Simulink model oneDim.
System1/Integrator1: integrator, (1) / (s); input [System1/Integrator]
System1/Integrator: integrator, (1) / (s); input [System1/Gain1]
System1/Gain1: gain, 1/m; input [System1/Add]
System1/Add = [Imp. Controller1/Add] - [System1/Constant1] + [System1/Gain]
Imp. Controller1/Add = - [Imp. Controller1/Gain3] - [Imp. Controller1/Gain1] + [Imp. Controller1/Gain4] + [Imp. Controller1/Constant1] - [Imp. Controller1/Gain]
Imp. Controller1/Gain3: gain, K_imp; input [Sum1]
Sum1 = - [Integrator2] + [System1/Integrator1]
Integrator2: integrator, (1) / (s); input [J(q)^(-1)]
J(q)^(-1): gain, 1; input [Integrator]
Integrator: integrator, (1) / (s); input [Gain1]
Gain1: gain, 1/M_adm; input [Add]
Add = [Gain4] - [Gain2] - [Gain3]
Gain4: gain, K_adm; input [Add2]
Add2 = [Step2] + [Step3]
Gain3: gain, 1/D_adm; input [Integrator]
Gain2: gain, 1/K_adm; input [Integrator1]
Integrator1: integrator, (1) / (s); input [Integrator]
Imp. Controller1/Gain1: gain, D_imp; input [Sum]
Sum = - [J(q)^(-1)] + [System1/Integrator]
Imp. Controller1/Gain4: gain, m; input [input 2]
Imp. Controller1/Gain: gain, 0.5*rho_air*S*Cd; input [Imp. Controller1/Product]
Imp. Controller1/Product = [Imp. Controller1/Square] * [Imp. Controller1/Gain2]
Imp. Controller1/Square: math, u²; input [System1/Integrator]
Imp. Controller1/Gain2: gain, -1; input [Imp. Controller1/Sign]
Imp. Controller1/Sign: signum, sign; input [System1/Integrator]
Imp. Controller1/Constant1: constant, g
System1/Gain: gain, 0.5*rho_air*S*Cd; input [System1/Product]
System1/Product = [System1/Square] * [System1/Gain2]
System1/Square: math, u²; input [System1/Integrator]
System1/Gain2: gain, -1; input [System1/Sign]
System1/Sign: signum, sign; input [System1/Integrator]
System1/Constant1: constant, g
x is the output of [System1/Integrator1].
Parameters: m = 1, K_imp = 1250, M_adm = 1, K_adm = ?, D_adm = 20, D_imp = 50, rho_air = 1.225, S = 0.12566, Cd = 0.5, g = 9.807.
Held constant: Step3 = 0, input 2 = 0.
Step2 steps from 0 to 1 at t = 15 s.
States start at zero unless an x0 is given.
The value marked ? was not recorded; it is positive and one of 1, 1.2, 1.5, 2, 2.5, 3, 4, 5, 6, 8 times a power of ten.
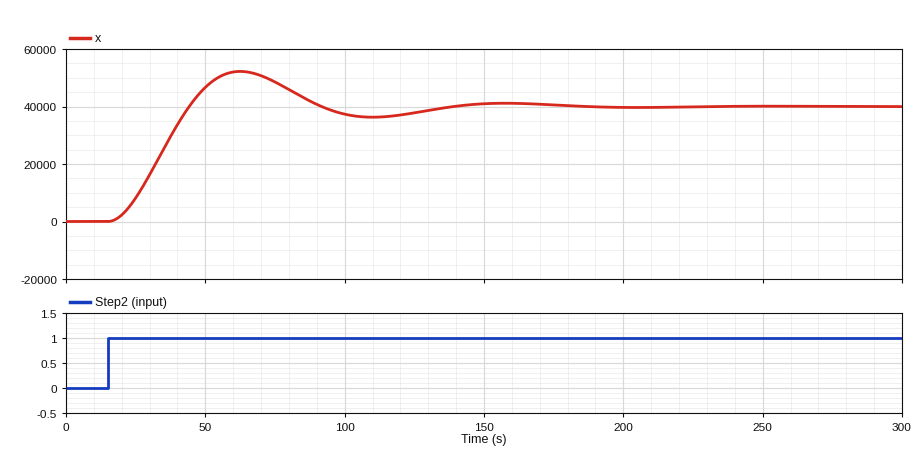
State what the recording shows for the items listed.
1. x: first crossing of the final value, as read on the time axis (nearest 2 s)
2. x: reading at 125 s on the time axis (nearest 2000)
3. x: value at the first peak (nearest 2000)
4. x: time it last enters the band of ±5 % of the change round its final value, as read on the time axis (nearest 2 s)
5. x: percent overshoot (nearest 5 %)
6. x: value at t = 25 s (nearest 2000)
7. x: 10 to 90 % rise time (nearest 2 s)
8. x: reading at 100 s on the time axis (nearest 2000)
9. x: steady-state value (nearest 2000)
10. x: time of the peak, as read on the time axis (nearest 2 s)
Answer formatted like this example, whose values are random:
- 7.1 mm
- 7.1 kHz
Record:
- 44 s
- 38000
- 52000
- 126 s
- 30 %
- 8000
- 20 s
- 38000
- 40000
- 62 s
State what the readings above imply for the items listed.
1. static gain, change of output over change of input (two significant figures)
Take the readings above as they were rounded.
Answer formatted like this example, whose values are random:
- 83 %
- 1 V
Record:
- 40000
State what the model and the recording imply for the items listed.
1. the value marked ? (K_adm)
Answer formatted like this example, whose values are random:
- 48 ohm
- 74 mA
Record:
- 200
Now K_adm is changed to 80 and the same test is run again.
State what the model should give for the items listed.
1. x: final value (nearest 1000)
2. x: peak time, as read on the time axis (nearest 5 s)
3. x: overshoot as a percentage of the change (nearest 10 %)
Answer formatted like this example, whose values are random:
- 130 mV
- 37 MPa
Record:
- 6000
- 45 s
- 50 %
